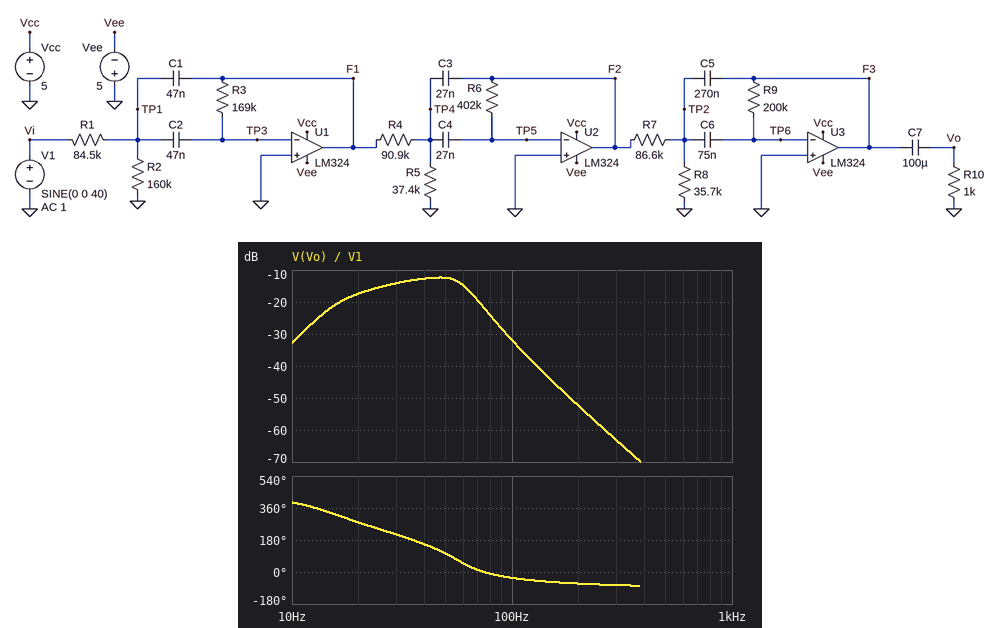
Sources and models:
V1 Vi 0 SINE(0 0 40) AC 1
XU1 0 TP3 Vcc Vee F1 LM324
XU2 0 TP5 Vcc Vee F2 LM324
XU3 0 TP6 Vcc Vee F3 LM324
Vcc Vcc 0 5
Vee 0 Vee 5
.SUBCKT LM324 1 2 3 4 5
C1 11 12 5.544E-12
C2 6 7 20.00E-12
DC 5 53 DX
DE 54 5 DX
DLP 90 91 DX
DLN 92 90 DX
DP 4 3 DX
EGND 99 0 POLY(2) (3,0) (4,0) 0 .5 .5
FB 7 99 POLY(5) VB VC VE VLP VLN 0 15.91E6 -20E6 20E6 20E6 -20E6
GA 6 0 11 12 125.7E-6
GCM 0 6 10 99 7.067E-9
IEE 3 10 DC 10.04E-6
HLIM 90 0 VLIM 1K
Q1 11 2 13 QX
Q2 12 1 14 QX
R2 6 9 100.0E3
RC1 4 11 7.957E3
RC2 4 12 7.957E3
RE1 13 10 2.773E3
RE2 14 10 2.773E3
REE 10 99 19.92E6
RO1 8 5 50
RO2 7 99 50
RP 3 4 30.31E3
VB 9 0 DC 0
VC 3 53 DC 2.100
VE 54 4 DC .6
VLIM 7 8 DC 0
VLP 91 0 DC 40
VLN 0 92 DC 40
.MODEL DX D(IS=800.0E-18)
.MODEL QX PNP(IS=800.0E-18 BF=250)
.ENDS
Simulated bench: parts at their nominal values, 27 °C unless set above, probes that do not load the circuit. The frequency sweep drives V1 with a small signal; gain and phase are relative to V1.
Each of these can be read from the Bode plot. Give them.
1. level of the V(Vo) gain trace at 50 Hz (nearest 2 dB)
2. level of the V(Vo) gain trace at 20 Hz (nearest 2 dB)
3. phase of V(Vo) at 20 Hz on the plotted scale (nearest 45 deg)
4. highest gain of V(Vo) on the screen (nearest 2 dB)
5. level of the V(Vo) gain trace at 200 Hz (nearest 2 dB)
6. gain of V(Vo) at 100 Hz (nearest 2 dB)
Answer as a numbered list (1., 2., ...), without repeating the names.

1. -12 dB
2. -18 dB
3. 270 deg
4. -12 dB
5. -52 dB
6. -32 dB
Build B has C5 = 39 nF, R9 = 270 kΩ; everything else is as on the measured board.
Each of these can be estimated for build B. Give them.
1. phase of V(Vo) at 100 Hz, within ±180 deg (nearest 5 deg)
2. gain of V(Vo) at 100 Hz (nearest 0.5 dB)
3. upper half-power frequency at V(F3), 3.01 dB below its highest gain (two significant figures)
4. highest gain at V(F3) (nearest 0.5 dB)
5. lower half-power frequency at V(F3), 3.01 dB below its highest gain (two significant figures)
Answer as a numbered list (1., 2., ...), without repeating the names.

1. -25 deg
2. -14.5 dB
3. 59 Hz
4. 8.0 dB
5. 33 Hz
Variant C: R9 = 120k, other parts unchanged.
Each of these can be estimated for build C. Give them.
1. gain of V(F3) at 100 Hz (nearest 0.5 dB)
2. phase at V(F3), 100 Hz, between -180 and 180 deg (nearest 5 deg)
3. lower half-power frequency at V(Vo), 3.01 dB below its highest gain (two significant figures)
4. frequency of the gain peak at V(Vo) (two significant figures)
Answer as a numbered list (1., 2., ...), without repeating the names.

1. -32.0 dB
2. -30 deg
3. 28 Hz
4. 48 Hz
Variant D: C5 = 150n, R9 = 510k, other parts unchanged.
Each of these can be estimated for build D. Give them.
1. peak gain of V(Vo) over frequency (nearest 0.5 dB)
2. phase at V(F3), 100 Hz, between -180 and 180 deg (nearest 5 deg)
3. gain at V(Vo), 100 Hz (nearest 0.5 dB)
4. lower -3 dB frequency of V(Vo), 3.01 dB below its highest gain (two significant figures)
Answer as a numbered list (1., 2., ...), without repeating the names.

1. -7.0 dB
2. -40 deg
3. -27.0 dB
4. 23 Hz
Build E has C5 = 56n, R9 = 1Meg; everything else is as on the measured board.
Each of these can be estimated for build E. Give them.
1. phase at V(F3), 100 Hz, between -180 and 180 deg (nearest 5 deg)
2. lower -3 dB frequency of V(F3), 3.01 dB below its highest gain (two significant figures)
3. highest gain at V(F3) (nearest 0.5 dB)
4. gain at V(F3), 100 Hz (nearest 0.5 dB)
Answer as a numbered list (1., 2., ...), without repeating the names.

1. -40 deg
2. 14 Hz
3. 2.0 dB
4. -18.0 dB
